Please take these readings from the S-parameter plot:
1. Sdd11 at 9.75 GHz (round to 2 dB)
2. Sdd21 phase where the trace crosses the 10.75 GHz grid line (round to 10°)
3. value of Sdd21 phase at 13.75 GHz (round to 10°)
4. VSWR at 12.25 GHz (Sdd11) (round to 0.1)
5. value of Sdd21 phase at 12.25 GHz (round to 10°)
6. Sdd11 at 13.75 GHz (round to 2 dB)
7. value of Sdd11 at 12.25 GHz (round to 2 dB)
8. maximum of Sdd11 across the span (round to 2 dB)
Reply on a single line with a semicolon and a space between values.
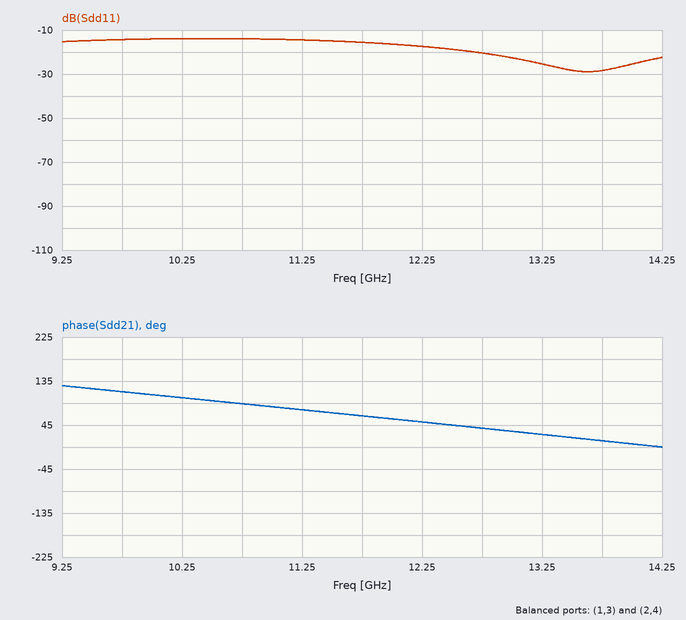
-14 dB; 90°; 10°; 1.3; 50°; -28 dB; -18 dB; -14 dB
